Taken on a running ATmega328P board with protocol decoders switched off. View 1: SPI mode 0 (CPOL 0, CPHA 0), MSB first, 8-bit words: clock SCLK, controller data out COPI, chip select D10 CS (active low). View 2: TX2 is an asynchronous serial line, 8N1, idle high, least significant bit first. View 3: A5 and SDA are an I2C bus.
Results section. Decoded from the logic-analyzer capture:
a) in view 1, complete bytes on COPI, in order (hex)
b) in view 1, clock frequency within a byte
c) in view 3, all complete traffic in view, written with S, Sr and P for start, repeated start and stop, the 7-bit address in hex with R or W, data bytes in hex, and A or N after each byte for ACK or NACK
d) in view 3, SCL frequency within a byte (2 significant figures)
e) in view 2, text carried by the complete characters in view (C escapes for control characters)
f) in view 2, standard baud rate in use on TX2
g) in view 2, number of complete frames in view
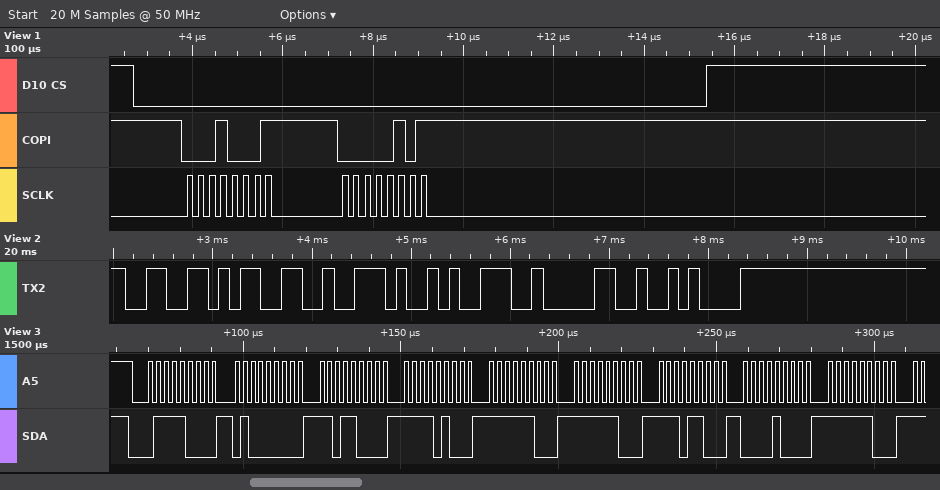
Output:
0x11 0x05
4 MHz
S 3CW A 40 A D8 A F4 A FC A FC A EC A 08 A FC A
400 kHz
"f3.90\n"
9600 baud
6
